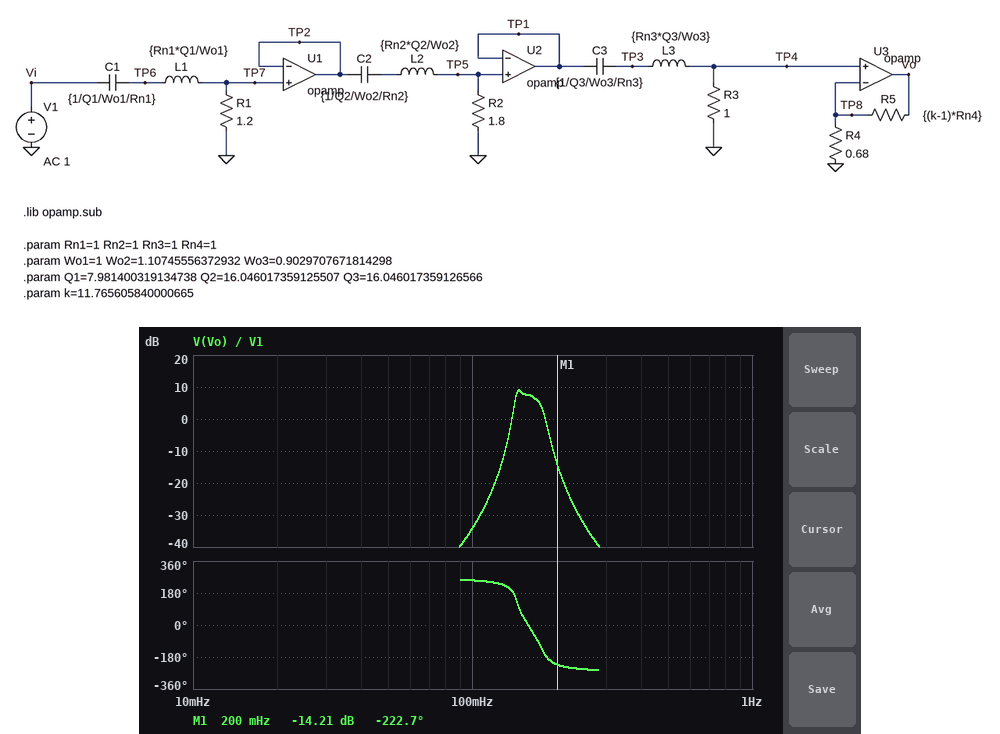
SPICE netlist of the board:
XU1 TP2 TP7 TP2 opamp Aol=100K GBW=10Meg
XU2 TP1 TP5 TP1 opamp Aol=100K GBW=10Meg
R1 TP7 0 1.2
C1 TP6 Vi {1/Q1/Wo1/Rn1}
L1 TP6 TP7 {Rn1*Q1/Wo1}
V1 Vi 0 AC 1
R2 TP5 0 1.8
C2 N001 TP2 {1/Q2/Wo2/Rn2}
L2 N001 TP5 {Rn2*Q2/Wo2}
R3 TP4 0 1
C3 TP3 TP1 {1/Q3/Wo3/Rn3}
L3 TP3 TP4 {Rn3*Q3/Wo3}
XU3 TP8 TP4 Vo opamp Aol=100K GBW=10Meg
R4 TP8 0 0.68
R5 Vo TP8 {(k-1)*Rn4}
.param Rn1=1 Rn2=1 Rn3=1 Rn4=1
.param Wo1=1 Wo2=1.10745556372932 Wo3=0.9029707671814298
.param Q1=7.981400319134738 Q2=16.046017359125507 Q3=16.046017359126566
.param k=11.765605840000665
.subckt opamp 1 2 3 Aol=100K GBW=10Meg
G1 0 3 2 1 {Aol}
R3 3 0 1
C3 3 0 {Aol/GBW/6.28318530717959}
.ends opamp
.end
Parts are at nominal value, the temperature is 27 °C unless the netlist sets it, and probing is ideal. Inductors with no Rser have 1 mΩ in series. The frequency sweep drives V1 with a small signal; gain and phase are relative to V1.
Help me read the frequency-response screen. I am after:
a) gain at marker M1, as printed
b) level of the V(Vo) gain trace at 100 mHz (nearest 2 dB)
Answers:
-14.21 dB
-34 dB
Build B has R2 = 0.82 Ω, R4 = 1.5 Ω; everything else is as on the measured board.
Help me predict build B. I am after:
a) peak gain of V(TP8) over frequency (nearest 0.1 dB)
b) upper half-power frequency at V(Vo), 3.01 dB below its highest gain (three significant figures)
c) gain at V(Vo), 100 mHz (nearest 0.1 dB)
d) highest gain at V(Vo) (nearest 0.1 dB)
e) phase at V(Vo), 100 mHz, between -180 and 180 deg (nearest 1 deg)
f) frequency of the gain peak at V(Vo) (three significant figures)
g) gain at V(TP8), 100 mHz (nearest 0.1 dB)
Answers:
-20.7 dB
179 mHz
-46.9 dB
-2.4 dB
-106 deg
175 mHz
-65.2 dB
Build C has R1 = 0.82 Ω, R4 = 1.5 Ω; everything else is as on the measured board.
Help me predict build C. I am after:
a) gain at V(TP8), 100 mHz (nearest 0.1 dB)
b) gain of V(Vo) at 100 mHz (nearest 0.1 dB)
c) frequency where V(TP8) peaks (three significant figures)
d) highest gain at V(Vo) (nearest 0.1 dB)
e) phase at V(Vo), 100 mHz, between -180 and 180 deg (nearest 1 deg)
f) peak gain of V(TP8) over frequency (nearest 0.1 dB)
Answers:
-61.6 dB
-43.4 dB
158 mHz
1.2 dB
-106 deg
-17.0 dB
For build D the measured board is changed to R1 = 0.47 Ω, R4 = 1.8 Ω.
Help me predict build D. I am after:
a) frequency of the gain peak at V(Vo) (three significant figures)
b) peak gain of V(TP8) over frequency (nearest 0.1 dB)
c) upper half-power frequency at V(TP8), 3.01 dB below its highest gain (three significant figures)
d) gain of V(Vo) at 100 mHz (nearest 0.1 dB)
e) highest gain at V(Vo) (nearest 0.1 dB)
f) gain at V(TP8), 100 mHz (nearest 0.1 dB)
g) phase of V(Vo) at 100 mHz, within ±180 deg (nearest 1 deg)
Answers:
159 mHz
-17.1 dB
164 mHz
-49.5 dB
-0.2 dB
-66.4 dB
-104 deg
